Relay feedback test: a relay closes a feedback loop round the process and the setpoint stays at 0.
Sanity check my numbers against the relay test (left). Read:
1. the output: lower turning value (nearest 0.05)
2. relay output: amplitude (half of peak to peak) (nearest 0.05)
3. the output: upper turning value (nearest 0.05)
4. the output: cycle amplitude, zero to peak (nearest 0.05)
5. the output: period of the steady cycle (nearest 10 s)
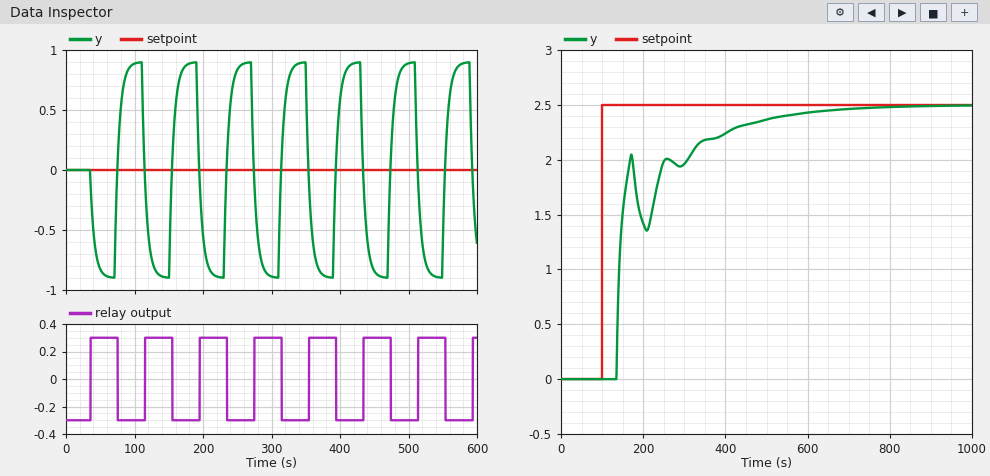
-0.90
0.30
0.90
0.90
80 s
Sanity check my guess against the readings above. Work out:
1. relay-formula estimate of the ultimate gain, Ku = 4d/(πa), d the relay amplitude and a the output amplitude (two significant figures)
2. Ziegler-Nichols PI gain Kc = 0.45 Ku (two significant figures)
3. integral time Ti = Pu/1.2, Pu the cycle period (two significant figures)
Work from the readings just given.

0.42
0.19
67 s
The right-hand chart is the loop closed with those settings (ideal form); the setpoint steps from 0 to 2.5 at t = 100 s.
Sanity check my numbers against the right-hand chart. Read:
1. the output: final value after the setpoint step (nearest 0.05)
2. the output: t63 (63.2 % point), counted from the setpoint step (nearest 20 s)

2.50
60 s
